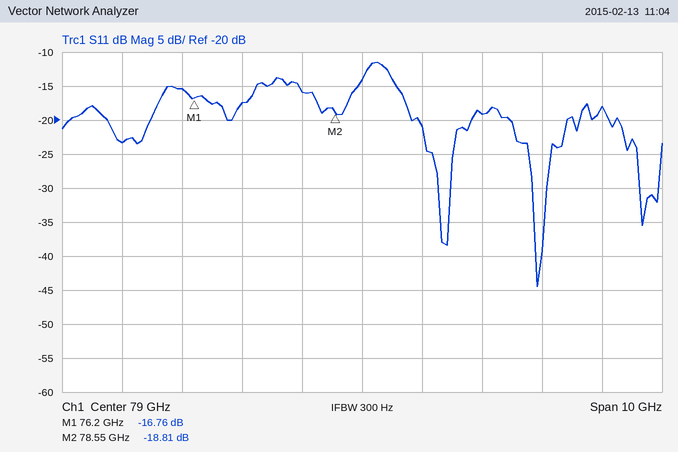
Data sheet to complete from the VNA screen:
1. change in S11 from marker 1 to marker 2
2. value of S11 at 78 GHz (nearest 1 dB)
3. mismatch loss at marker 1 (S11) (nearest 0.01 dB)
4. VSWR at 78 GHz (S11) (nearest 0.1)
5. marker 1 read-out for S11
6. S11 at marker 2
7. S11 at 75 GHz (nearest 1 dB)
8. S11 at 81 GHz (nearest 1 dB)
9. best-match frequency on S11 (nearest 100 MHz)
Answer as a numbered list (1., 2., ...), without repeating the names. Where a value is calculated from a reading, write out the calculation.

1. -18.81 − (-16.76) = -2.05 dB
2. -16 dB
3. −10 log10(1 − 10^(-16.76/10)) ≈ 0.09 dB
4. |Γ| = 10^(-16/20) = 0.1585; VSWR = (1 + 0.1585)/(1 − 0.1585) ≈ 1.4
5. -16.76 dB
6. -18.81 dB
7. -23 dB
8. -19 dB
9. 81.9 GHz
